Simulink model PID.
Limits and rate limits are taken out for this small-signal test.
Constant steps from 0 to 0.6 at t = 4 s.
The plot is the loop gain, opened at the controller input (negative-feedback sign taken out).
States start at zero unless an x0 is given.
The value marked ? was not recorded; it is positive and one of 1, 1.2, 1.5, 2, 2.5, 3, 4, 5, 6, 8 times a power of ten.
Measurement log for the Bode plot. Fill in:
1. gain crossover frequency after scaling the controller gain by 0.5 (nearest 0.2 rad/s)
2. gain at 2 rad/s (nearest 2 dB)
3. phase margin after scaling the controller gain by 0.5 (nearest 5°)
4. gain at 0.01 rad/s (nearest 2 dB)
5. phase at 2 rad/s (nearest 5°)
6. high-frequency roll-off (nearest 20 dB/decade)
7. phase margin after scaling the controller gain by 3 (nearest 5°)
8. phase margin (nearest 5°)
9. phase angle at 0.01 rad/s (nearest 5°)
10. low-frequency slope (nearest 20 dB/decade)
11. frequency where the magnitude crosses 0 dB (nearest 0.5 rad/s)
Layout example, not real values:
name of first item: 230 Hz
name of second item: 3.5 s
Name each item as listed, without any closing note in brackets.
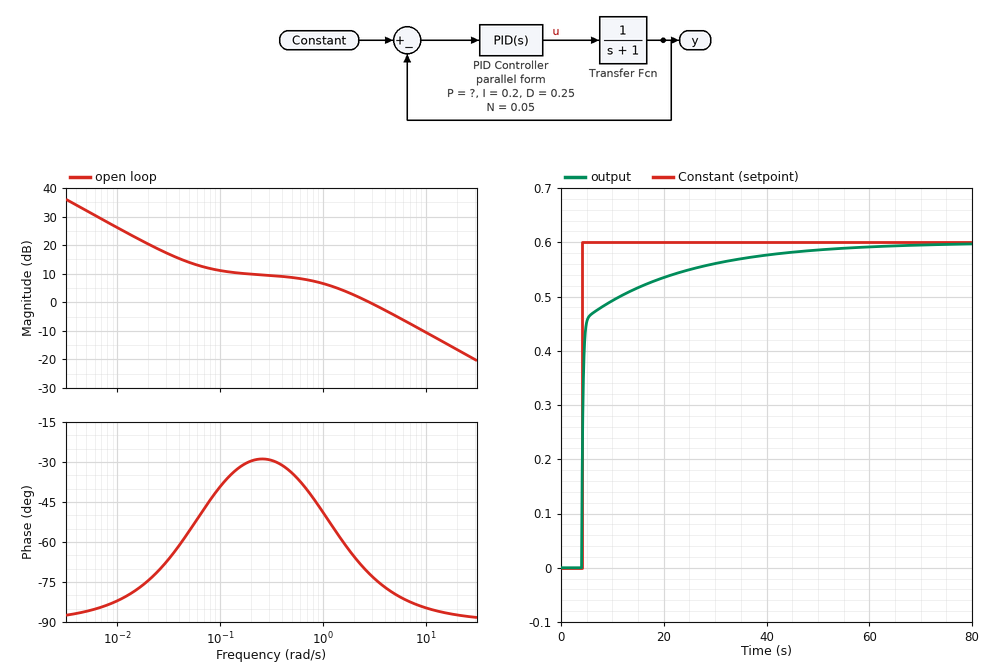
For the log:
gain crossover frequency after scaling the controller gain by 0.5: 1.2 rad/s
gain at 2 rad/s: 2 dB
phase margin after scaling the controller gain by 0.5: 130°
gain at 0.01 rad/s: 26 dB
phase at 2 rad/s: -65°
high-frequency roll-off: -20 dB/decade
phase margin after scaling the controller gain by 3: 95°
phase margin: 110°
phase angle at 0.01 rad/s: -80°
low-frequency slope: -20 dB/decade
frequency where the magnitude crosses 0 dB: 3.0 rad/s
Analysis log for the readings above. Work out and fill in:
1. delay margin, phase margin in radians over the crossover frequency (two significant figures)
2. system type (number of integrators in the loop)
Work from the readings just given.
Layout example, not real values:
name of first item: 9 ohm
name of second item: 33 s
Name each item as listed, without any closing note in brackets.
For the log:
delay margin, phase margin in radians over the crossover frequency: 0.64 s
system type: 1
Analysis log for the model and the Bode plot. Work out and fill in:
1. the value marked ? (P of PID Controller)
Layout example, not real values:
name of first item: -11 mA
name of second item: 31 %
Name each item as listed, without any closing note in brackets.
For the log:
the value marked ?: 3
